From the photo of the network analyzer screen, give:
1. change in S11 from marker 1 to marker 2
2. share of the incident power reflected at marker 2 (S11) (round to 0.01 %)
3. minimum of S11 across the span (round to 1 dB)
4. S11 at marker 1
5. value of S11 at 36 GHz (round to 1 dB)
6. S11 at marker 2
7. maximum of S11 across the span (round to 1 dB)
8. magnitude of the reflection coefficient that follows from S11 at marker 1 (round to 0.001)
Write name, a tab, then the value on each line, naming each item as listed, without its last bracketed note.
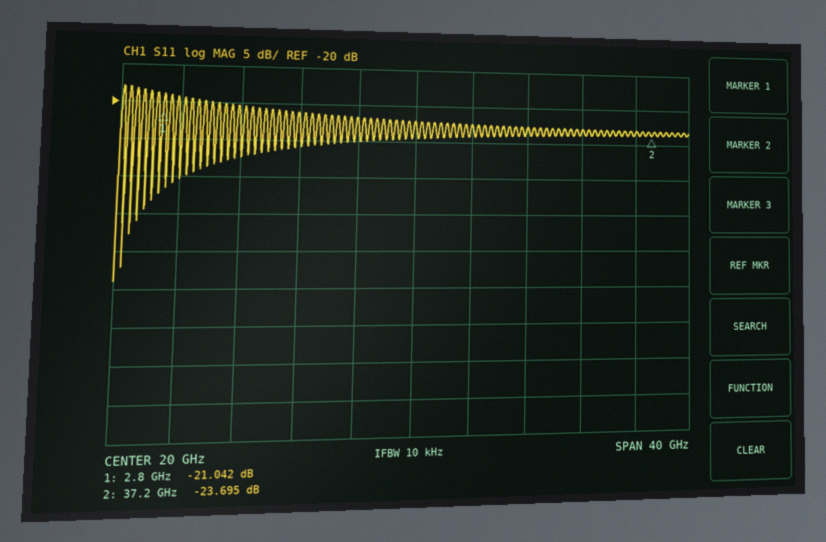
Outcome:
change in S11 from marker 1 to marker 2	-2.653 dB
share of the incident power reflected at marker 2 (S11)	0.43 %
minimum of S11 across the span	-44 dB
S11 at marker 1	-21.042 dB
value of S11 at 36 GHz	-23 dB
S11 at marker 2	-23.695 dB
maximum of S11 across the span	-18 dB
magnitude of the reflection coefficient that follows from S11 at marker 1	0.089
